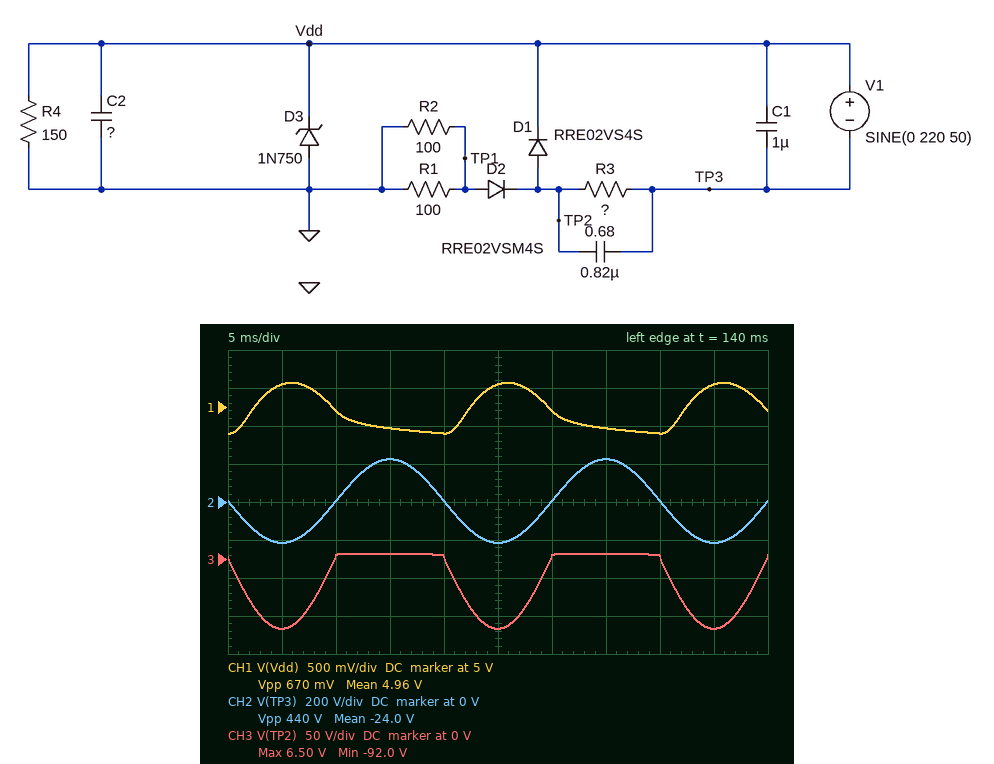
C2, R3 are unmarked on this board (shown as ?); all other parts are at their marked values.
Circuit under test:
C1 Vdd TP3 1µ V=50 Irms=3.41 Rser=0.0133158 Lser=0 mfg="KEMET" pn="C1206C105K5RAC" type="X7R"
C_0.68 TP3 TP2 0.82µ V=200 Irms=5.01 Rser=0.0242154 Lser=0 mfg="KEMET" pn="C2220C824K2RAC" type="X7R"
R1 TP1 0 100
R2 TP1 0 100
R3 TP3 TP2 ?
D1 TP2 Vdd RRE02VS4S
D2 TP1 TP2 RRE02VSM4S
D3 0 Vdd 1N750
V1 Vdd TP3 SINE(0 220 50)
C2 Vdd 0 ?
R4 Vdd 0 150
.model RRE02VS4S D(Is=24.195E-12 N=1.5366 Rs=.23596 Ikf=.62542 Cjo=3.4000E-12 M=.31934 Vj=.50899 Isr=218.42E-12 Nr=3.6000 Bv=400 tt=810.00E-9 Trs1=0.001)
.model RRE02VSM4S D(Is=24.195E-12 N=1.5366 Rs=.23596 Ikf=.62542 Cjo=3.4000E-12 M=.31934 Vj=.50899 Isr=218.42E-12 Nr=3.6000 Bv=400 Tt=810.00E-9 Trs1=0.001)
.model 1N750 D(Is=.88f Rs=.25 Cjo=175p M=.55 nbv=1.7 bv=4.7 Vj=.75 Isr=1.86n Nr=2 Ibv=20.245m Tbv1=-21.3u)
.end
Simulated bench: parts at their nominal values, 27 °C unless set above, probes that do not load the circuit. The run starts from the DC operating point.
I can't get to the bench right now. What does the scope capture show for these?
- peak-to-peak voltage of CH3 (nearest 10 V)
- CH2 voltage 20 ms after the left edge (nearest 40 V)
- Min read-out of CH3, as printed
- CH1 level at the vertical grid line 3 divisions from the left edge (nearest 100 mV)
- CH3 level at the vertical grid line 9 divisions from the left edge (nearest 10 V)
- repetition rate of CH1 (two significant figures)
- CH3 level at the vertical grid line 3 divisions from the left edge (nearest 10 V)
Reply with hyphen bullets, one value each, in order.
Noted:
- 100 V
- 0 V
- -92.0 V
- 4.7 V
- -90 V
- 50 Hz
- 10 V
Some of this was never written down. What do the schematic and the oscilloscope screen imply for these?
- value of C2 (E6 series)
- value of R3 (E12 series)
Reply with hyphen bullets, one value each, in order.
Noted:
- 3.3 mF
- 68 Ω
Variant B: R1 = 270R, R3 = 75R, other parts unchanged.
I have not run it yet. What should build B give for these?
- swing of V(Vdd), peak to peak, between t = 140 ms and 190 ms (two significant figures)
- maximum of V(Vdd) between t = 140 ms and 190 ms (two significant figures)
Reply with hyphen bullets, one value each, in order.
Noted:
- 570 mV
- 5.2 V
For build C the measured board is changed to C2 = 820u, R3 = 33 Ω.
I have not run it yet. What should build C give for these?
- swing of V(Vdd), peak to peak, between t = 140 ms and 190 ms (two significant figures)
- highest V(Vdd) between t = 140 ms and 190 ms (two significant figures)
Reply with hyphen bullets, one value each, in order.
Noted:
- 1.2 V
- 5.5 V
